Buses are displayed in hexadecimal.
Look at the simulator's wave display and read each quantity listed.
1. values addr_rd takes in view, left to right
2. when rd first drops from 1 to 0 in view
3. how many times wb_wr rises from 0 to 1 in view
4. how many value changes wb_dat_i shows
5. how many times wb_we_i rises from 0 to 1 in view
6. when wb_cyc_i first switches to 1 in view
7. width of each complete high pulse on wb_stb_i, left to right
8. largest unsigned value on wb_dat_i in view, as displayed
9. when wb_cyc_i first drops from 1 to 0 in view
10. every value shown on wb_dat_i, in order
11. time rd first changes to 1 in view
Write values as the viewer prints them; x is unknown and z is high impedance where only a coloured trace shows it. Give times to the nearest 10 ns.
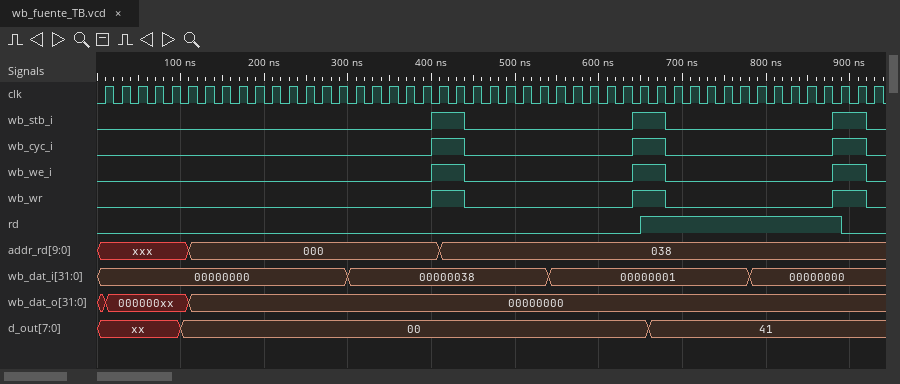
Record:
xxx, 000, 038
890 ns
3
3
3
400 ns
40 ns, 40 ns, 40 ns
00000038
440 ns
00000000, 00000038, 00000001, 00000000
650 ns
